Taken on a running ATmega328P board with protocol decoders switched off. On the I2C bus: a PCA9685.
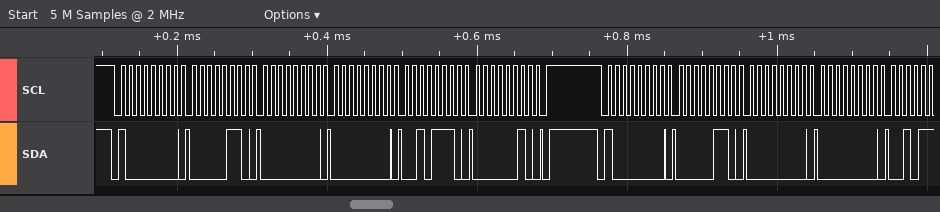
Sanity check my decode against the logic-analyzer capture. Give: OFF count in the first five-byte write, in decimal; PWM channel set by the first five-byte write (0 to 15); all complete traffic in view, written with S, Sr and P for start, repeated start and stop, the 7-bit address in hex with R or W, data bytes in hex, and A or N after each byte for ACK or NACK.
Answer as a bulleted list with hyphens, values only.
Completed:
- 558
- 0
- S 40W A 06 A 00 A 00 A 2E A 02 A P S 40W A 06 A 00 A 00 A
